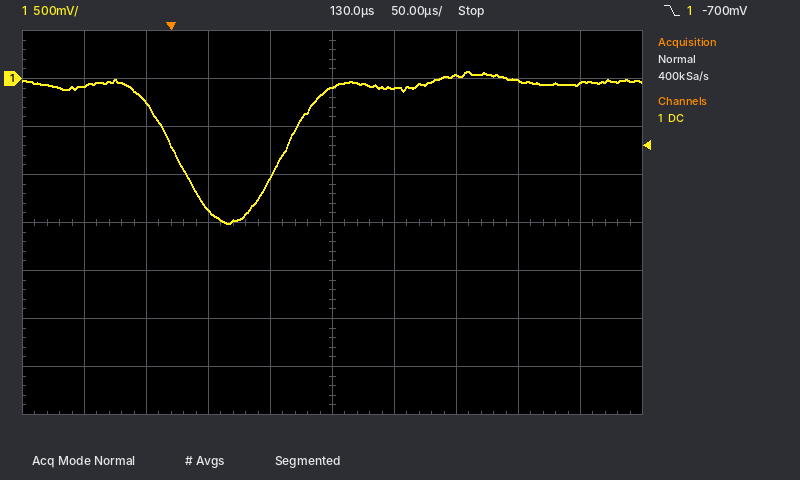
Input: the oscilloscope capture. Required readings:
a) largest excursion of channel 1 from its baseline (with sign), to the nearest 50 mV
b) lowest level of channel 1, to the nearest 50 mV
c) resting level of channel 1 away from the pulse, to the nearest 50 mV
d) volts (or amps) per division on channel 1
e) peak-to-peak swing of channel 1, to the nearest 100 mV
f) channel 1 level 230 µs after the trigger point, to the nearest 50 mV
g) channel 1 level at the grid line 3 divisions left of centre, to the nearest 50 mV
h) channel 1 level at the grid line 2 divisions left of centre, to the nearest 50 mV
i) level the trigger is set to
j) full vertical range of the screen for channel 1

-1.45 V
-1.50 V
-50 mV
500 mV
1.60 V
50 mV
-250 mV
-1.35 V
-700 mV
4 V
